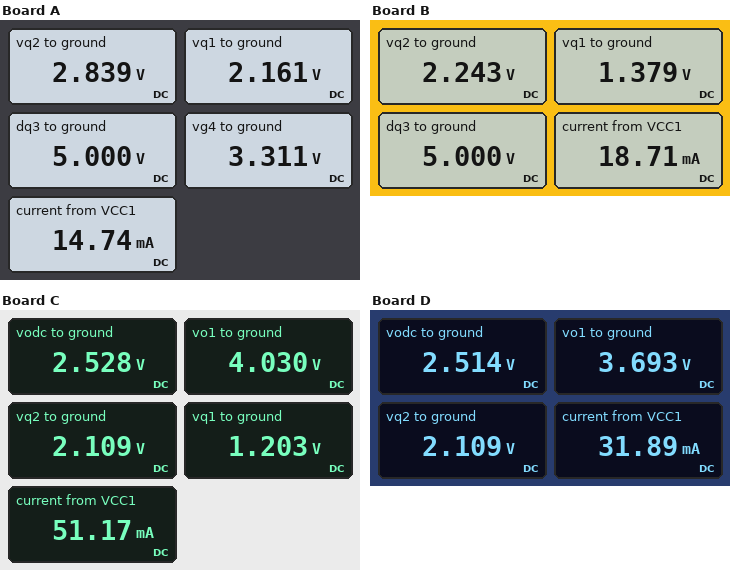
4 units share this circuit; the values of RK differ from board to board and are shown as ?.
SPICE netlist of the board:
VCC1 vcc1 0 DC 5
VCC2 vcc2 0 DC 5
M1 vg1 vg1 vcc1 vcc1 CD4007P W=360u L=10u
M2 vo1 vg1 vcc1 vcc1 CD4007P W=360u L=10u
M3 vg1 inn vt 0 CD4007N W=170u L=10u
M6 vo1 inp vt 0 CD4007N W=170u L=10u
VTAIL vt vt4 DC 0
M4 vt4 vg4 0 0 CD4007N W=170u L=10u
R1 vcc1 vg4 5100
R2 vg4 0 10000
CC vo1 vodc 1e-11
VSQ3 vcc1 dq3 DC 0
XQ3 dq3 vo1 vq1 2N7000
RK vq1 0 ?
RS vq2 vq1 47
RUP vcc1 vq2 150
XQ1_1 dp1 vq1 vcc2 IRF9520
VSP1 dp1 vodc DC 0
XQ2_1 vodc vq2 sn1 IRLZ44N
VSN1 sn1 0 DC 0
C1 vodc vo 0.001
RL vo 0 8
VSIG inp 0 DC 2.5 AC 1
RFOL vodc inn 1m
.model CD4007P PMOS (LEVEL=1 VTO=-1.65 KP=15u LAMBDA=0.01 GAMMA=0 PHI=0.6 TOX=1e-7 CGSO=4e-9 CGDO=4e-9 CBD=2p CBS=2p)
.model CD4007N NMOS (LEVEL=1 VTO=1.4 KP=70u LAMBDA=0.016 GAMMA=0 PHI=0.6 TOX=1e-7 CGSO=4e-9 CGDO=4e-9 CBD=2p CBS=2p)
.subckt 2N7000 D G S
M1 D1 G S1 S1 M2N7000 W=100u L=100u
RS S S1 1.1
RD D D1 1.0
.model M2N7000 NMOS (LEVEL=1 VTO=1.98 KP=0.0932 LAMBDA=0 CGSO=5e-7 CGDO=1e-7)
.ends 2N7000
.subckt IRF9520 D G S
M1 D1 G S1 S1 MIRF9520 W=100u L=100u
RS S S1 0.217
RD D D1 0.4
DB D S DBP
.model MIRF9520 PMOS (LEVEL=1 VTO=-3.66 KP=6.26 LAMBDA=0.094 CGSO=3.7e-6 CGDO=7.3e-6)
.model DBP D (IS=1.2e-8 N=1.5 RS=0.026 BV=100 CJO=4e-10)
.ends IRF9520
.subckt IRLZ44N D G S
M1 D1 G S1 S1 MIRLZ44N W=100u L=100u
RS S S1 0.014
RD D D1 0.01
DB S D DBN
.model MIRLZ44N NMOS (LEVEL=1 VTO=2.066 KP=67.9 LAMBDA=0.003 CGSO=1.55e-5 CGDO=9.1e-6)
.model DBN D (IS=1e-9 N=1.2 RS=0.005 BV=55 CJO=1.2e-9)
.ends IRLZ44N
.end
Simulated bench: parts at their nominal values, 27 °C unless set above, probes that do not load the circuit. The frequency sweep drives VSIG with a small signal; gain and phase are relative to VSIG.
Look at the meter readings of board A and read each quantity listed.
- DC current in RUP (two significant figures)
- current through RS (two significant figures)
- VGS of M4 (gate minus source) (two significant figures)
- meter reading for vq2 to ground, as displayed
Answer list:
14 mA
14 mA
3.3 V
2.839 V
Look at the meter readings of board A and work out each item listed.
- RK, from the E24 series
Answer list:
150 Ω
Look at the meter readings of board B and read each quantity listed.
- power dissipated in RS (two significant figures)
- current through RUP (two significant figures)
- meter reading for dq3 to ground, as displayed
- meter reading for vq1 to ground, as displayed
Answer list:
16 mW
18 mA
5.000 V
1.379 V
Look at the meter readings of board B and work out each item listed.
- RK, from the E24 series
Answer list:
75 Ω
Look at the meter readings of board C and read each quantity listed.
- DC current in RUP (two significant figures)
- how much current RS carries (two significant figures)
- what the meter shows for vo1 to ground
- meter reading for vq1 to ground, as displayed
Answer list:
19 mA
19 mA
4.030 V
1.203 V
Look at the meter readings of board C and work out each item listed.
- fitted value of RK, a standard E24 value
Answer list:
24 Ω
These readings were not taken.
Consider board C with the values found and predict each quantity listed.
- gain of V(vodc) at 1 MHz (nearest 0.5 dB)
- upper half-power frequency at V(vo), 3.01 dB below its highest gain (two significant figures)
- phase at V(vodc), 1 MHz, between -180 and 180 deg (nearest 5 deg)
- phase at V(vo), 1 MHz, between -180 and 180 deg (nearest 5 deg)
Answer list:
2.5 dB
2.5 MHz
-10 deg
-10 deg
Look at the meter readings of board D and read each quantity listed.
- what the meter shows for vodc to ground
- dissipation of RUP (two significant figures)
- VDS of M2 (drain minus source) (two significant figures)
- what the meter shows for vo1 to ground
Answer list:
2.514 V
56 mW
-1.3 V
3.693 V
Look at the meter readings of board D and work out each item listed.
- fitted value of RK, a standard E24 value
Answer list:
39 Ω
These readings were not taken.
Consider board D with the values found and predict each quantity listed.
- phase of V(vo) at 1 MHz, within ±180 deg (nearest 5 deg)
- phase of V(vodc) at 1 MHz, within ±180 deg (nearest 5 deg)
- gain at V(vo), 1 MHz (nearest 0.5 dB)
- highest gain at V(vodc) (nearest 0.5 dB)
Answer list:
-5 deg
-5 deg
2.5 dB
21.5 dB
